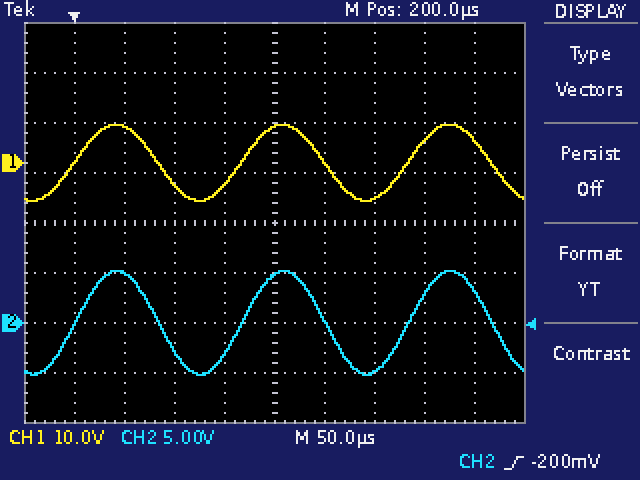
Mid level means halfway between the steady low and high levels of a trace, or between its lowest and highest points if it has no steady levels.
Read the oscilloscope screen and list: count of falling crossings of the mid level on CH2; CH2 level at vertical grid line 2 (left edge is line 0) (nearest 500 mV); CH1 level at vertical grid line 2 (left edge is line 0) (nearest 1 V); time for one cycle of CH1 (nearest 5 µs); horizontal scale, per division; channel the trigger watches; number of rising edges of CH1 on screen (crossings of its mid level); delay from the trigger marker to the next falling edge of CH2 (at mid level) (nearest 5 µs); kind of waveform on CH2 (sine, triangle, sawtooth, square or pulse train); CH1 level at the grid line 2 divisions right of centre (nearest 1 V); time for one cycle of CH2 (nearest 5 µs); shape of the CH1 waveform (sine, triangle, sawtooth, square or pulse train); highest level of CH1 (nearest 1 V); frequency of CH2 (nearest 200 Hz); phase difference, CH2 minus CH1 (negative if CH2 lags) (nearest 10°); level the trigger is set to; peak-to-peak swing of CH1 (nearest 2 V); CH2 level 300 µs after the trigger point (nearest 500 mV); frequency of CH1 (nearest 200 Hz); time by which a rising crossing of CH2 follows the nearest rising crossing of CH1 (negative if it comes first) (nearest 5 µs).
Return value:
3
5.0 V
7 V
165 µs
50 µs
CH2
3
85 µs
sine
-7 V
165 µs
sine
8 V
6.0 kHz
0°
-200 mV
16 V
-5.0 V
6.0 kHz
0 µs
